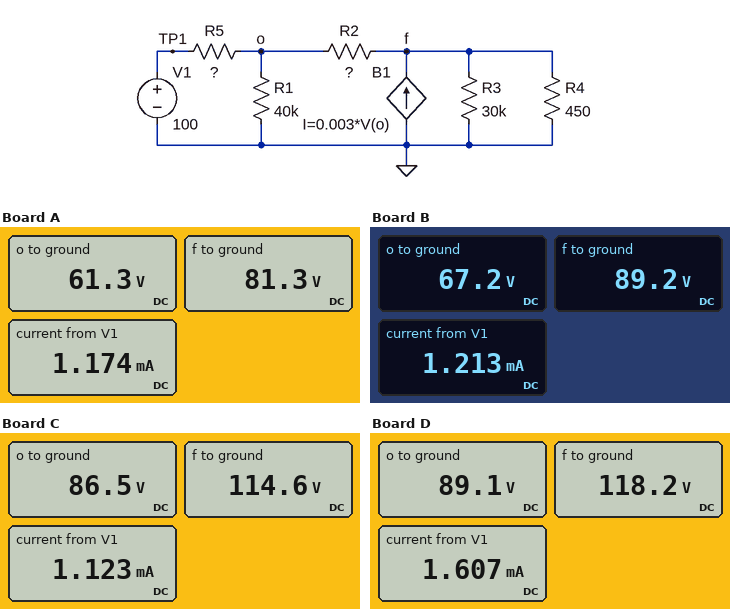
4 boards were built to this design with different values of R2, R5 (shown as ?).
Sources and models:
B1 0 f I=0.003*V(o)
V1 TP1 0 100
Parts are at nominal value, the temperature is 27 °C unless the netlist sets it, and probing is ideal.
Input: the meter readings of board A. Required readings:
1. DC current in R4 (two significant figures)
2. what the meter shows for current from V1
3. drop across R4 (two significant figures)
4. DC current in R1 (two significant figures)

180 mA
1.174 mA
81 V
1.5 mA
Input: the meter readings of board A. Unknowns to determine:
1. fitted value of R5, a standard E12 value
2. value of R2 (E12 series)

33 kΩ
56 kΩ
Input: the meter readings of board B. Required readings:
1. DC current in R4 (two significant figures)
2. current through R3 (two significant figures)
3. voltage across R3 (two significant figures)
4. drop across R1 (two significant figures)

200 mA
3.0 mA
89 V
67 V
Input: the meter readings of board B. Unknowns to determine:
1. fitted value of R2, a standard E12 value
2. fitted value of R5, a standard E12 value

47 kΩ
27 kΩ
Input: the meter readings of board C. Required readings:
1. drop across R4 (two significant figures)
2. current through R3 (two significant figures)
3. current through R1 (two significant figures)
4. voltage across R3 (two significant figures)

110 V
3.8 mA
2.2 mA
110 V
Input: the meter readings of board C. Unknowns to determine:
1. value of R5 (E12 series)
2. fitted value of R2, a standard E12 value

12 kΩ
27 kΩ
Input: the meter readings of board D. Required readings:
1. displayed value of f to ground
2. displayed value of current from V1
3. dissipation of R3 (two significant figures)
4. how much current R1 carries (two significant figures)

118.2 V
1.607 mA
470 mW
2.2 mA
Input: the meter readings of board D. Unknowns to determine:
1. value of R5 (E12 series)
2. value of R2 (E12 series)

6.8 kΩ
47 kΩ
